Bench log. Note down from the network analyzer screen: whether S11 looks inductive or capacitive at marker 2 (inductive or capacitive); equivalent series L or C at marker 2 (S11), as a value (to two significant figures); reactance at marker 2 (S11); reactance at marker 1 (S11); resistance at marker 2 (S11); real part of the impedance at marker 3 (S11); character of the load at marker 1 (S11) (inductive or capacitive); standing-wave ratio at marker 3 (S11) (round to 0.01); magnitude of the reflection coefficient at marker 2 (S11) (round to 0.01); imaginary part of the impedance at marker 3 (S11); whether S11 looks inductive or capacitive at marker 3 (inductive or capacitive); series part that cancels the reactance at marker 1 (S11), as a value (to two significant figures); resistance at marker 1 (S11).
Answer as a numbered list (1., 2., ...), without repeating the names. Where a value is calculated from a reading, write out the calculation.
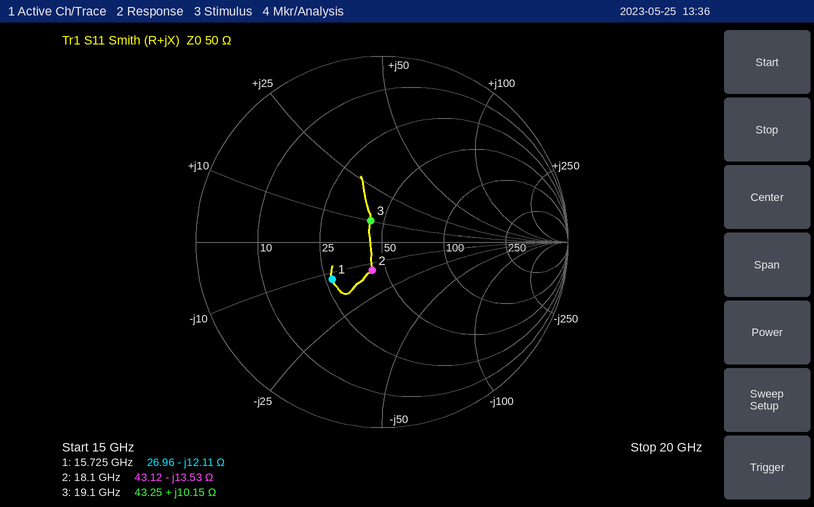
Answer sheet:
1. capacitive
2. C = 1/(2π × 18.1 GHz × 13.53 Ω) ≈ 650 fF
3. -13.53 Ω
4. -12.11 Ω
5. 43.12 Ω
6. 43.25 Ω
7. capacitive
8. 1.30
9. 0.16
10. +10.15 Ω
11. inductive
12. L = 12.11 Ω/(2π × 15.725 GHz) ≈ 123 pH, so 120 pH to two significant figures
13. 26.96 Ω
